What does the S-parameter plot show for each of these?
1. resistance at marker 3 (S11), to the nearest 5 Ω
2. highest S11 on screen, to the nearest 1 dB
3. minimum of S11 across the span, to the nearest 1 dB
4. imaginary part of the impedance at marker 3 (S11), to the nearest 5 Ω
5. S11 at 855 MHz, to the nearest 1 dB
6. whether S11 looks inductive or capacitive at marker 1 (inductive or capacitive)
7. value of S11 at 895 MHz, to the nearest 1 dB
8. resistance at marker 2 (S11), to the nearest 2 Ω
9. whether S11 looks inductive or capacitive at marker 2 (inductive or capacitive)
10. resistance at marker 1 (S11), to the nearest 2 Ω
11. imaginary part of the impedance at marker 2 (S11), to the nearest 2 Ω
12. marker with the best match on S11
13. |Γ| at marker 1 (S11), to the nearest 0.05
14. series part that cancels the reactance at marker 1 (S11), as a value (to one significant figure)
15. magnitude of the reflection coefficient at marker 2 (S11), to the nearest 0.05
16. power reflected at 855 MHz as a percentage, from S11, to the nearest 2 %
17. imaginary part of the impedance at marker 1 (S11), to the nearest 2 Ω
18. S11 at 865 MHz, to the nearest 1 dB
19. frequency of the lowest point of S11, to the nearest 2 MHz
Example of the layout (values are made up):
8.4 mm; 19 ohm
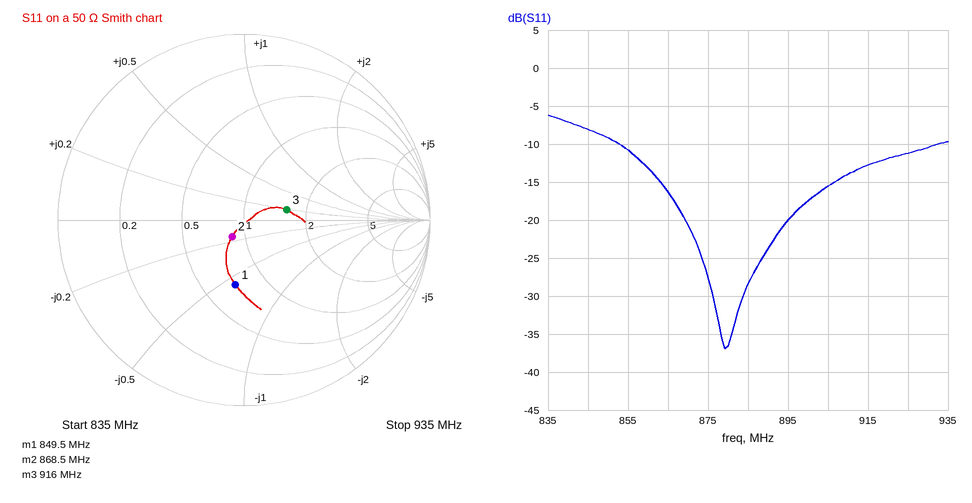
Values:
80 Ω; -6 dB; -37 dB; +10 Ω; -11 dB; capacitive; -20 dB; 44 Ω; capacitive; 36 Ω; -8 Ω; marker 2; 0.35; 5 nH; 0.10; 8 %; -28 Ω; -16 dB; 880 MHz
